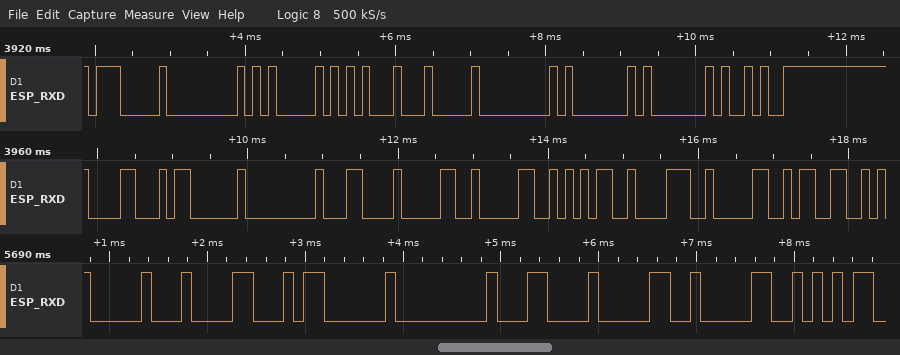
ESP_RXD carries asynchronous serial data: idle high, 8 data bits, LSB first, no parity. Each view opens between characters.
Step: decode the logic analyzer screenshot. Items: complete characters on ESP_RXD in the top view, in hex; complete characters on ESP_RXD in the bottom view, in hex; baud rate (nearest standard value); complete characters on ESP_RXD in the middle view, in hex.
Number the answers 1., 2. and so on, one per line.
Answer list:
1. 07, 00, 05, 15, 04, 00, 01, 01, 29
2. 10, 18, 03, 00, 0C, 30, 30
3. 9600 baud
4. 18, 03, 00, 0C, 30, 30, 35, 38, 30, 33
